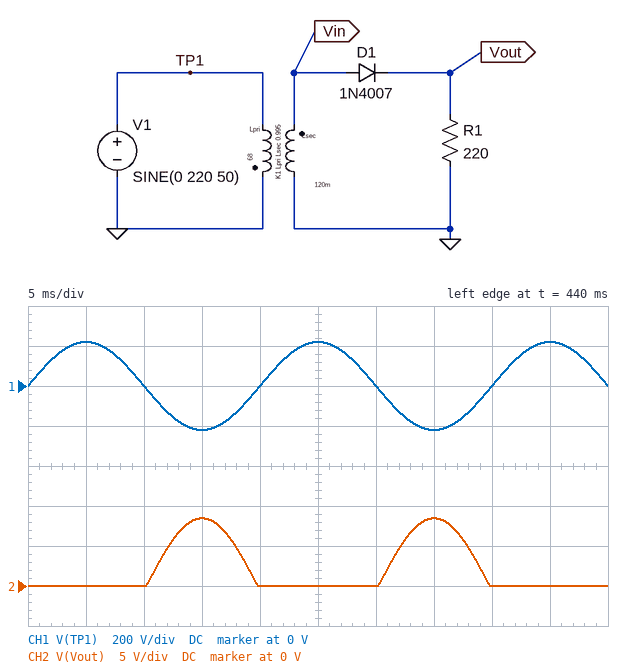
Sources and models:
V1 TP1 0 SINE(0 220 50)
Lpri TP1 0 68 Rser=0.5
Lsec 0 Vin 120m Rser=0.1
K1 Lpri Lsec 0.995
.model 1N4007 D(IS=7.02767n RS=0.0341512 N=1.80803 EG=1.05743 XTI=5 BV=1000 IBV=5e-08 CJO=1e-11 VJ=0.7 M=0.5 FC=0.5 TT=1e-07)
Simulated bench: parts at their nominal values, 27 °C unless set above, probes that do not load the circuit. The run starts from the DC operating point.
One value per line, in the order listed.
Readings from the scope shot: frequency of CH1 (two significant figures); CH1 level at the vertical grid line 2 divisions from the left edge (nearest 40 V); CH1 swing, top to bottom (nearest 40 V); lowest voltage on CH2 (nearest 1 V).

50 Hz
0 V
440 V
0 V
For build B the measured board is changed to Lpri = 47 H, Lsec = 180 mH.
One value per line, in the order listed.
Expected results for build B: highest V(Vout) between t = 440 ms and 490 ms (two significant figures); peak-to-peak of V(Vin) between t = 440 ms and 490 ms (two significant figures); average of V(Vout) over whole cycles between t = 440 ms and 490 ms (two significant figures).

13 V
27 V
4.0 V
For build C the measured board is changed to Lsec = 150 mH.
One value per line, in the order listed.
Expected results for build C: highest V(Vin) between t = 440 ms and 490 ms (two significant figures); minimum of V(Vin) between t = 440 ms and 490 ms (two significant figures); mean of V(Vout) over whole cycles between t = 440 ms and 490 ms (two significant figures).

10 V
-10 V
2.9 V
